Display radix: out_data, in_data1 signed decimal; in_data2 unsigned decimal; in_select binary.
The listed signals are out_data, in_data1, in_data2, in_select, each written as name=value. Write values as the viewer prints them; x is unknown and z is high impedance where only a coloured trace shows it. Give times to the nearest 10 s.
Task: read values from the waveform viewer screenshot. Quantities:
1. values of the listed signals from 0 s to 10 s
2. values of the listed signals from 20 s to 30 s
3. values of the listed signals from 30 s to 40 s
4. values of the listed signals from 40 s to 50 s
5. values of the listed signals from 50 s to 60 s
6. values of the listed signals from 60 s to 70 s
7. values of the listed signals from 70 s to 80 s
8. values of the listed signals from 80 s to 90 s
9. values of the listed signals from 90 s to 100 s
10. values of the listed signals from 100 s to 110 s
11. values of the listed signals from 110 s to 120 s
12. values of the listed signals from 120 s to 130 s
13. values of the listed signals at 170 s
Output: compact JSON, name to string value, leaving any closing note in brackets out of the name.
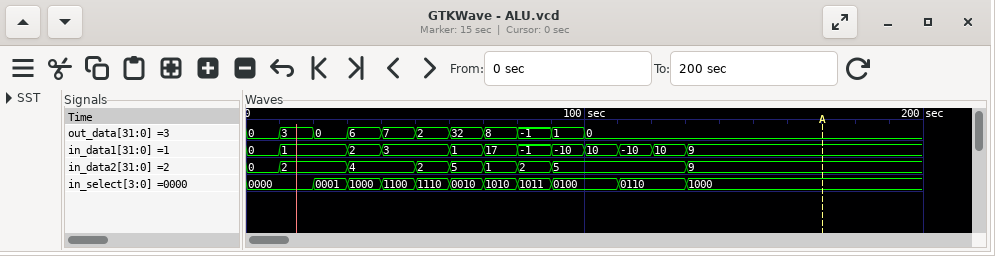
{"values of the listed signals from 0 s to 10 s": "out_data=0, in_data1=0, in_data2=0, in_select=0000", "values of the listed signals from 20 s to 30 s": "out_data=0, in_data1=1, in_data2=2, in_select=0001", "values of the listed signals from 30 s to 40 s": "out_data=6, in_data1=2, in_data2=4, in_select=1000", "values of the listed signals from 40 s to 50 s": "out_data=7, in_data1=3, in_data2=4, in_select=1100", "values of the listed signals from 50 s to 60 s": "out_data=2, in_data1=3, in_data2=2, in_select=1110", "values of the listed signals from 60 s to 70 s": "out_data=32, in_data1=1, in_data2=5, in_select=0010", "values of the listed signals from 70 s to 80 s": "out_data=8, in_data1=17, in_data2=1, in_select=1010", "values of the listed signals from 80 s to 90 s": "out_data=-1, in_data1=-1, in_data2=2, in_select=1011", "values of the listed signals from 90 s to 100 s": "out_data=1, in_data1=-10, in_data2=5, in_select=0100", "values of the listed signals from 100 s to 110 s": "out_data=0, in_data1=10, in_data2=5, in_select=0100", "values of the listed signals from 110 s to 120 s": "out_data=0, in_data1=-10, in_data2=5, in_select=0110", "values of the listed signals from 120 s to 130 s": "out_data=0, in_data1=10, in_data2=5, in_select=0110", "values of the listed signals at 170 s": "out_data=0, in_data1=9, in_data2=9, in_select=1000"}
